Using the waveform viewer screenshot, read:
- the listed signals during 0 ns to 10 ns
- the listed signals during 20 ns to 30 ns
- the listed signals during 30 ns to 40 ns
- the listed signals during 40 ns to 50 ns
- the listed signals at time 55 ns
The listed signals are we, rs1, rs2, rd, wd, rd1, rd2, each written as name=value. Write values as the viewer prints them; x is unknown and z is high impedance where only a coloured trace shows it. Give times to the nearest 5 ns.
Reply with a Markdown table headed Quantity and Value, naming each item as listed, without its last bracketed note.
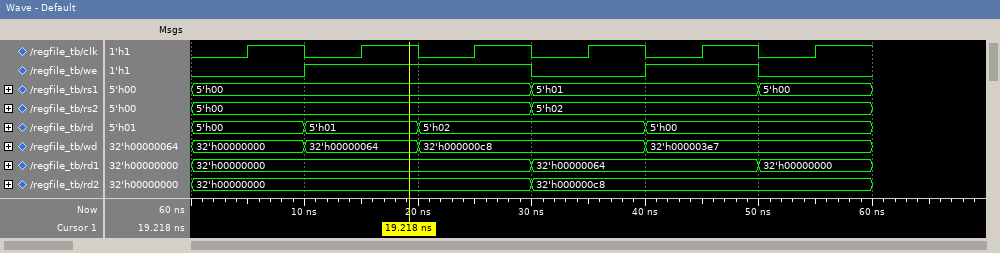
| Quantity | Value |
|---|---|
| the listed signals during 0 ns to 10 ns | we=0, rs1=5'h00, rs2=5'h00, rd=5'h00, wd=32'h00000000, rd1=32'h00000000, rd2=32'h00000000 |
| the listed signals during 20 ns to 30 ns | we=1, rs1=5'h00, rs2=5'h00, rd=5'h02, wd=32'h000000c8, rd1=32'h00000000, rd2=32'h00000000 |
| the listed signals during 30 ns to 40 ns | we=0, rs1=5'h01, rs2=5'h02, rd=5'h02, wd=32'h000000c8, rd1=32'h00000064, rd2=32'h000000c8 |
| the listed signals during 40 ns to 50 ns | we=1, rs1=5'h01, rs2=5'h02, rd=5'h00, wd=32'h000003e7, rd1=32'h00000064, rd2=32'h000000c8 |
| the listed signals at time 55 ns | we=0, rs1=5'h00, rs2=5'h02, rd=5'h00, wd=32'h000003e7, rd1=32'h00000000, rd2=32'h000000c8 |
